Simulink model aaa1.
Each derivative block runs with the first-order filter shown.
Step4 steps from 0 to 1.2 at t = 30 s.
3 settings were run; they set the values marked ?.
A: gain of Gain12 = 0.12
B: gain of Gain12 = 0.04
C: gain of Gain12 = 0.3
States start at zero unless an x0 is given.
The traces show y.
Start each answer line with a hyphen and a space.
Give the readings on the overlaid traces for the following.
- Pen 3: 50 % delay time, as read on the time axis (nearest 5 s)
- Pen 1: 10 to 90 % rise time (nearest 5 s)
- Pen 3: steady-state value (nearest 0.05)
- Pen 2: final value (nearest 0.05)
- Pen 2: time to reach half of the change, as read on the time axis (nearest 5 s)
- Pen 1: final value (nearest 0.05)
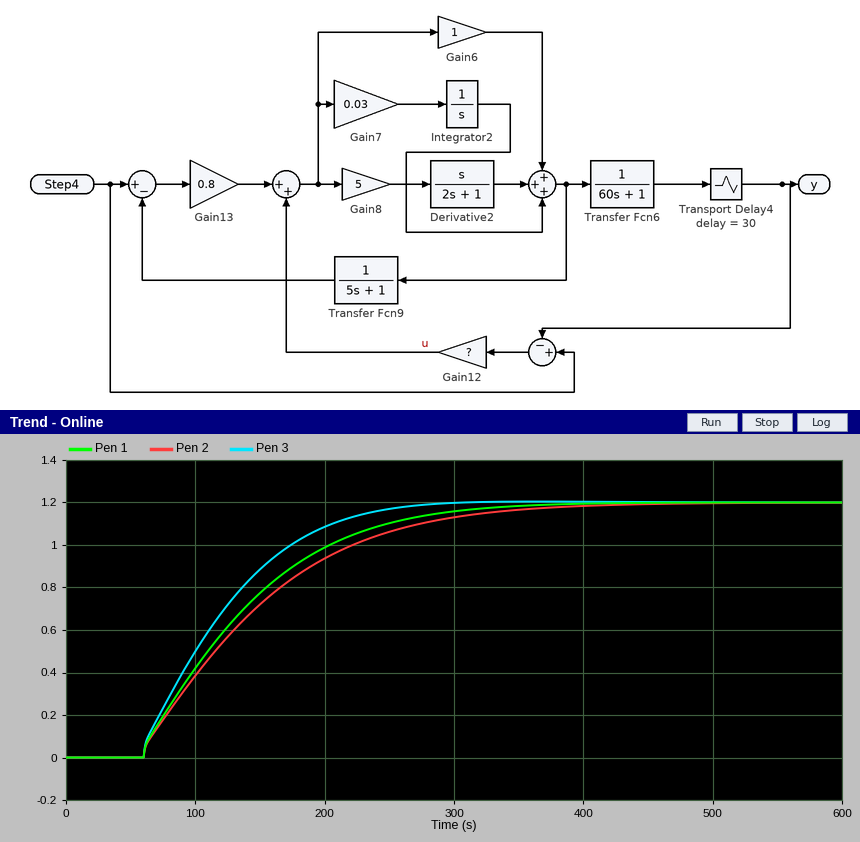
- 110 s
- 170 s
- 1.20
- 1.20
- 130 s
- 1.20
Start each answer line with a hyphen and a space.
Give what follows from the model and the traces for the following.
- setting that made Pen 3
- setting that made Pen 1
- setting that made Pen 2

- C
- A
- B
